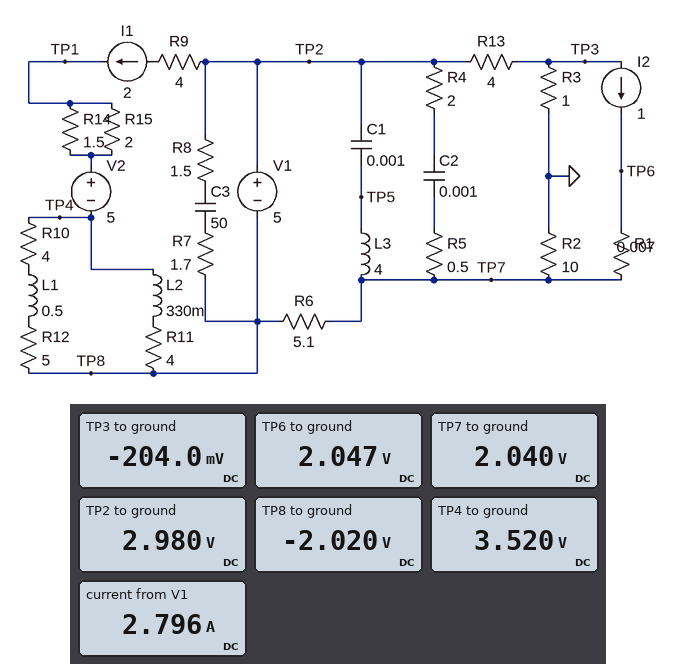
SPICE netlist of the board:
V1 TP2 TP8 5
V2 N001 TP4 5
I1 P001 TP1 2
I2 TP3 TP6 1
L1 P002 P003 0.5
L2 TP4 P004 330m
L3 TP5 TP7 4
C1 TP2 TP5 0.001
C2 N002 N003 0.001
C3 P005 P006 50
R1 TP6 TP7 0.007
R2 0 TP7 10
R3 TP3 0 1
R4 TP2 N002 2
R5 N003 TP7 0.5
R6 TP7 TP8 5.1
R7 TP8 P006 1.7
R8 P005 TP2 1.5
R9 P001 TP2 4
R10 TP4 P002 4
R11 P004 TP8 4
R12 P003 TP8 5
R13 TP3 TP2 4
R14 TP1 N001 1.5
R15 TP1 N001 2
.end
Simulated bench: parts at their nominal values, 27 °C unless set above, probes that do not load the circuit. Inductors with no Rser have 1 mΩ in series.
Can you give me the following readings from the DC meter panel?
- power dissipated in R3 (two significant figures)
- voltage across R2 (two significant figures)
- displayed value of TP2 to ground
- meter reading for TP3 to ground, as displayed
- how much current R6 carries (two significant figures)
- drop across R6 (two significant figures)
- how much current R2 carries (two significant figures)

42 mW
2.0 V
2.980 V
-204.0 mV
800 mA
4.1 V
200 mA
